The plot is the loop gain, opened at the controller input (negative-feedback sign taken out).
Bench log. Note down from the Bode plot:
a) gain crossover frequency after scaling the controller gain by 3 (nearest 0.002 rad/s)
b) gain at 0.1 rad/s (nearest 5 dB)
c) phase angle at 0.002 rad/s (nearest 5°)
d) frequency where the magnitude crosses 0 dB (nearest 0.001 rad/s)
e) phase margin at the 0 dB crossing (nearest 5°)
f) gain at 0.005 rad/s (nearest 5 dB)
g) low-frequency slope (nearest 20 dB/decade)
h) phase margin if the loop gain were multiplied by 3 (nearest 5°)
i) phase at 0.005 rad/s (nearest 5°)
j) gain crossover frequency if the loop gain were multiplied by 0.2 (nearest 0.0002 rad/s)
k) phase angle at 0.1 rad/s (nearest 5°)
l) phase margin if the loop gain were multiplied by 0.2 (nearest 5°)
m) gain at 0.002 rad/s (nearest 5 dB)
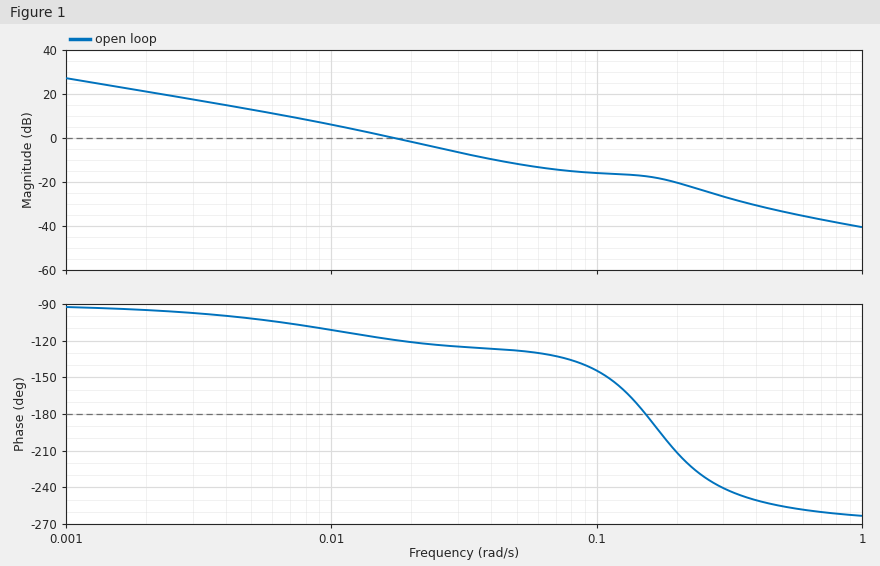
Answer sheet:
0.040 rad/s
-15 dB
-95°
0.017 rad/s
60°
15 dB
-20 dB/decade
55°
-100°
0.0044 rad/s
-145°
80°
20 dB
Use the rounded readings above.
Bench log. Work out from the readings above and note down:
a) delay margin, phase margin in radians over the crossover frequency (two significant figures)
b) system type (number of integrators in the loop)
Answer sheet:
62 s
1
